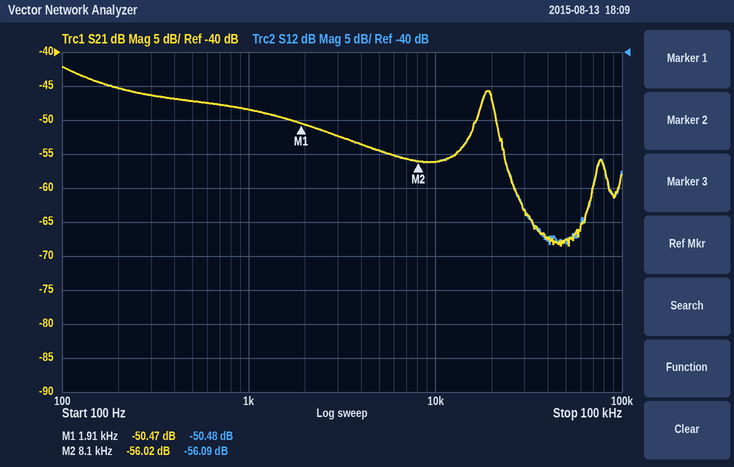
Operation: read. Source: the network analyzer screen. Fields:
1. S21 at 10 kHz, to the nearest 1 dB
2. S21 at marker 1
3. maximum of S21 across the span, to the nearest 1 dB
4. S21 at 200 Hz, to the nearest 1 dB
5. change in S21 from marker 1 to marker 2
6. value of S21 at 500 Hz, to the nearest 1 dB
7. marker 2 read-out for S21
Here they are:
-56 dB
-50.47 dB
-42 dB
-45 dB
-5.55 dB
-47 dB
-56.02 dB
